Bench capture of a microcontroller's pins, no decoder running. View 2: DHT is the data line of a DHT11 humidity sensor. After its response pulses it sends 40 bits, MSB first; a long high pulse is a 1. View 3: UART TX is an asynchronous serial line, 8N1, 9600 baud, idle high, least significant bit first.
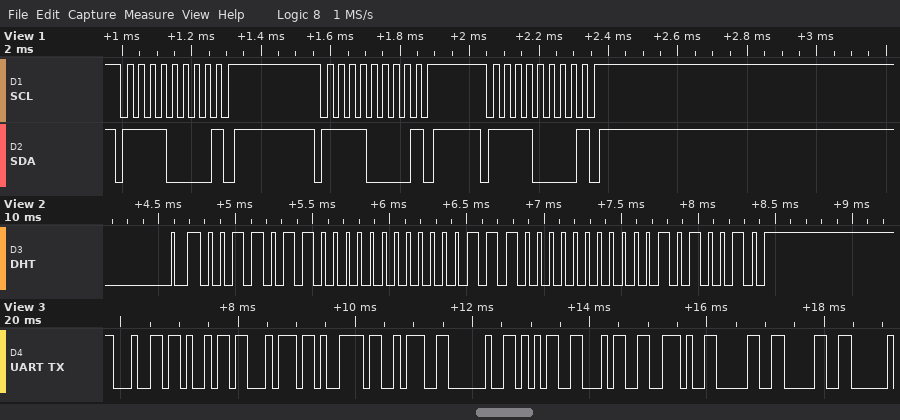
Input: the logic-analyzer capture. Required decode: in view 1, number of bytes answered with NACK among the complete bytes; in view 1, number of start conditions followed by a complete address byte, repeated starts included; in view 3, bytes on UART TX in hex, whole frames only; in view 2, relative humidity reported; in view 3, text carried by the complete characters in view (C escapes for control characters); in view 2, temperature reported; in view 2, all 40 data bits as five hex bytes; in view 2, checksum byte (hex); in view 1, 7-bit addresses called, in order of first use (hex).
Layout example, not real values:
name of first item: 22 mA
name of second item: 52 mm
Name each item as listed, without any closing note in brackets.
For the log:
in view 1, number of bytes answered with NACK among the complete bytes: 3
in view 1, number of start conditions followed by a complete address byte, repeated starts included: 3
in view 3, bytes on UART TX in hex, whole frames only: 64 69 74 79 3A 20 35 34 2E 30 30
in view 2, relative humidity reported: 54 %
in view 3, text carried by the complete characters in view: "dity: 54.00"
in view 2, temperature reported: 28.0 °C
in view 2, all 40 data bits as five hex bytes: 36 00 1C 00 52
in view 2, checksum byte: 0x52
in view 1, 7-bit addresses called, in order of first use: 0x78
